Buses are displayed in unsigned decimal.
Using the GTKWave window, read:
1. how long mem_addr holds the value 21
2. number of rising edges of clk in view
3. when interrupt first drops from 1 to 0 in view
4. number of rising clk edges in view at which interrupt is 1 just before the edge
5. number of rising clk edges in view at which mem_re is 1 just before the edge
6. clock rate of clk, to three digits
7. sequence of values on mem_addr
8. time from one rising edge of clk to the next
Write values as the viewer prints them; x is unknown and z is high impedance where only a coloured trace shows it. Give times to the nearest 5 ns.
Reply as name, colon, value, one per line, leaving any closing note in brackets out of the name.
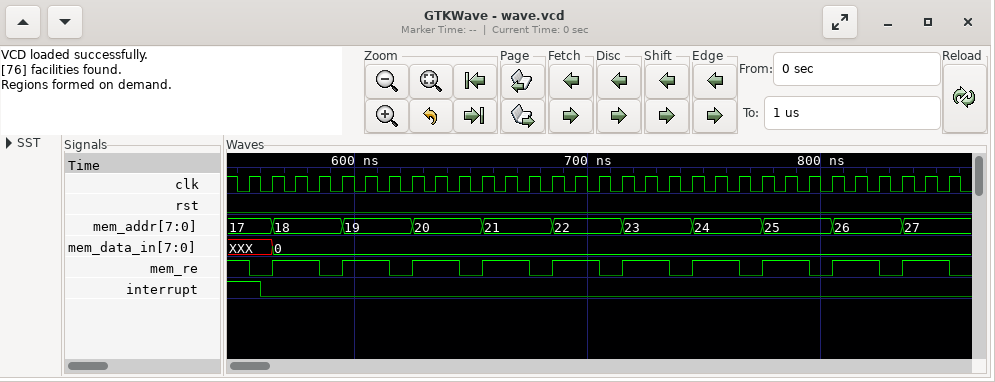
how long mem_addr holds the value 21: 30 ns
number of rising edges of clk in view: 31
when interrupt first drops from 1 to 0 in view: 560 ns
number of rising clk edges in view at which interrupt is 1 just before the edge: 1
number of rising clk edges in view at which mem_re is 1 just before the edge: 21
clock rate of clk, to three digits: 100 MHz
sequence of values on mem_addr: 17, 18, 19, 20, 21, 22, 23, 24, 25, 26, 27
time from one rising edge of clk to the next: 10 ns
